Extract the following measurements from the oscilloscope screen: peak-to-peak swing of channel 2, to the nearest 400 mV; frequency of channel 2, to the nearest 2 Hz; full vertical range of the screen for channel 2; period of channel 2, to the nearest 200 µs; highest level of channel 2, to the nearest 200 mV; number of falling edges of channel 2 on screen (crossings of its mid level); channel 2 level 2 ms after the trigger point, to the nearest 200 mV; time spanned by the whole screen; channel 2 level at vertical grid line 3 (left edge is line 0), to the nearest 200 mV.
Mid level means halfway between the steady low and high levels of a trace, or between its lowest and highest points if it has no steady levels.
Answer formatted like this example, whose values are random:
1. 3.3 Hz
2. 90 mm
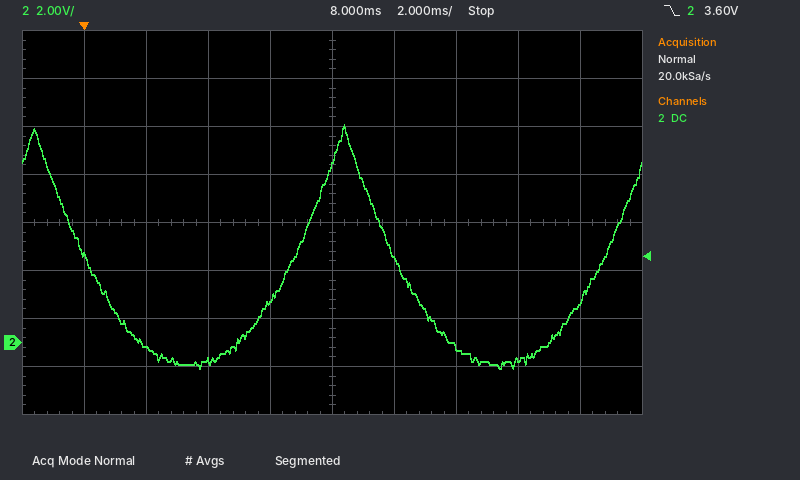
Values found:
1. 10.0 V
2. 100 Hz
3. 16 V
4. 10.0 ms
5. 9.0 V
6. 2
7. -200 mV
8. 20 ms
9. -800 mV
